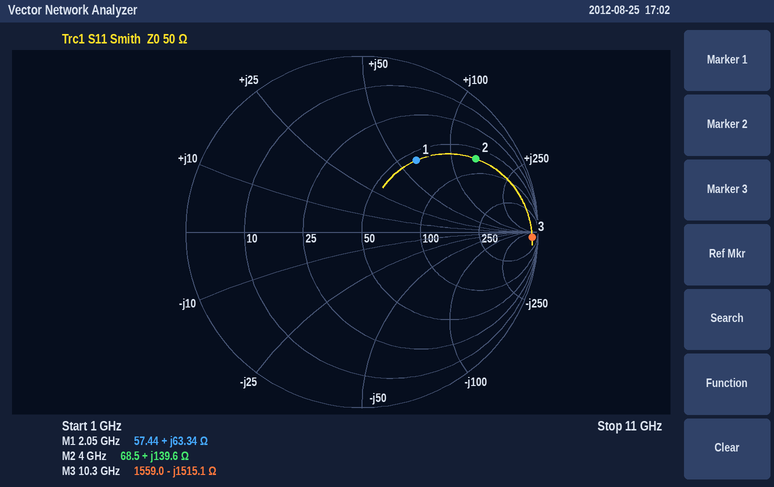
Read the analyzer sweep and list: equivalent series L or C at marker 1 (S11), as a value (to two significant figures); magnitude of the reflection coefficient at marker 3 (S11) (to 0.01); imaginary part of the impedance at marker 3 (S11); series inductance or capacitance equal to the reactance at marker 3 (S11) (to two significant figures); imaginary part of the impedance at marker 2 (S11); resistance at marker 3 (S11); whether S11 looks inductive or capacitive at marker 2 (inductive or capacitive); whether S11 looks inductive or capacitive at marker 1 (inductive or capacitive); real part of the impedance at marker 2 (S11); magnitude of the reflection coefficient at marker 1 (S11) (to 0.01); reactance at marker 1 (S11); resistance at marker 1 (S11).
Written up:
4.9 nH
0.97
-1515.1 Ω
10 fF
+139.6 Ω
1559.0 Ω
inductive
inductive
68.5 Ω
0.51
+63.34 Ω
57.44 Ω
